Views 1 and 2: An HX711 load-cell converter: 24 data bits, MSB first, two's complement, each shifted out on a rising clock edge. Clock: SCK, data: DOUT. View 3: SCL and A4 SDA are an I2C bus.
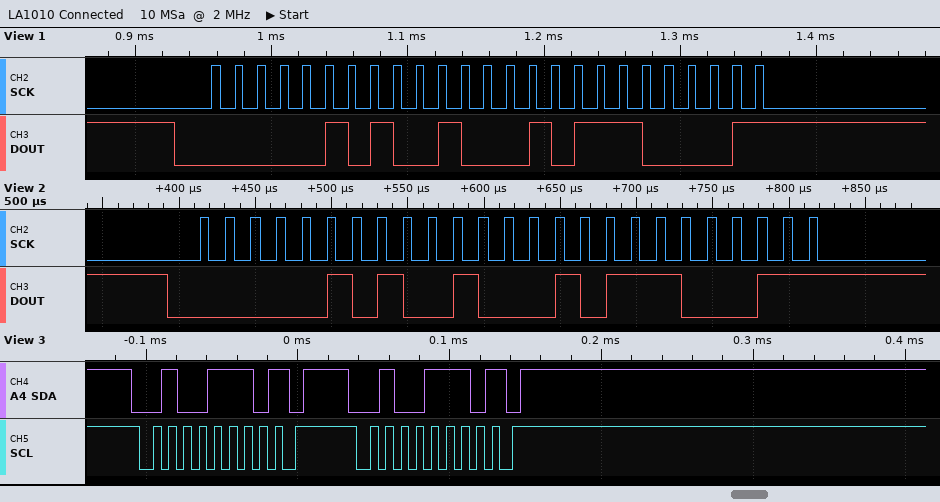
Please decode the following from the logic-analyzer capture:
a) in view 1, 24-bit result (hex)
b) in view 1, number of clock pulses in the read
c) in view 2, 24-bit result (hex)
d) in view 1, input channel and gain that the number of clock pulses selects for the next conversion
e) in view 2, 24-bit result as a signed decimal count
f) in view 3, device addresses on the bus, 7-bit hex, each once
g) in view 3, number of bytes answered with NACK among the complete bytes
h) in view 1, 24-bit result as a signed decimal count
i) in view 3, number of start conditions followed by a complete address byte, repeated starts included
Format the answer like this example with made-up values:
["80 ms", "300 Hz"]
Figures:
["0x0522E1", "25", "0x0522E3", "channel A, gain 128", "336611", "0x27", "2", "336609", "2"]
